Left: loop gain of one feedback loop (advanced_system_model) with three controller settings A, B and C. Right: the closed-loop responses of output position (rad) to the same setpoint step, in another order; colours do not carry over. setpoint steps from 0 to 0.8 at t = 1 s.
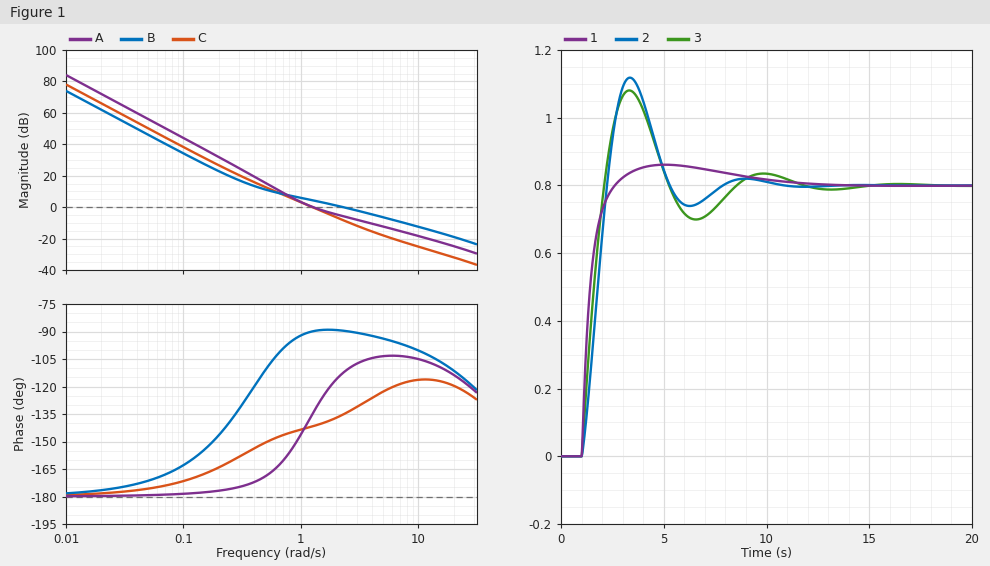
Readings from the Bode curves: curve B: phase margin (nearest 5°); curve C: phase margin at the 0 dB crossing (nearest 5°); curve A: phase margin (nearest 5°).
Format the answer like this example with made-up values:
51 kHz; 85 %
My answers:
90°; 40°; 45°
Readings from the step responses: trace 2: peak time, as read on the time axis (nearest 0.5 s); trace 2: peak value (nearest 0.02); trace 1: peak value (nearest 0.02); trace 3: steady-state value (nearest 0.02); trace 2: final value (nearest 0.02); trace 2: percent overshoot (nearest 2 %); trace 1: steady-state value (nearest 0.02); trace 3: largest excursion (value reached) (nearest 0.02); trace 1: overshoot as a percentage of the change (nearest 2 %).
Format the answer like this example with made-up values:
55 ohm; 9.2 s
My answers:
3.5 s; 1.12; 0.86; 0.80; 0.80; 40 %; 0.80; 1.08; 8 %
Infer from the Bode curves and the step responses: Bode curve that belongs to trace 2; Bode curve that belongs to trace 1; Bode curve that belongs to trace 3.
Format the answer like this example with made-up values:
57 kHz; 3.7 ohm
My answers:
C; B; A
